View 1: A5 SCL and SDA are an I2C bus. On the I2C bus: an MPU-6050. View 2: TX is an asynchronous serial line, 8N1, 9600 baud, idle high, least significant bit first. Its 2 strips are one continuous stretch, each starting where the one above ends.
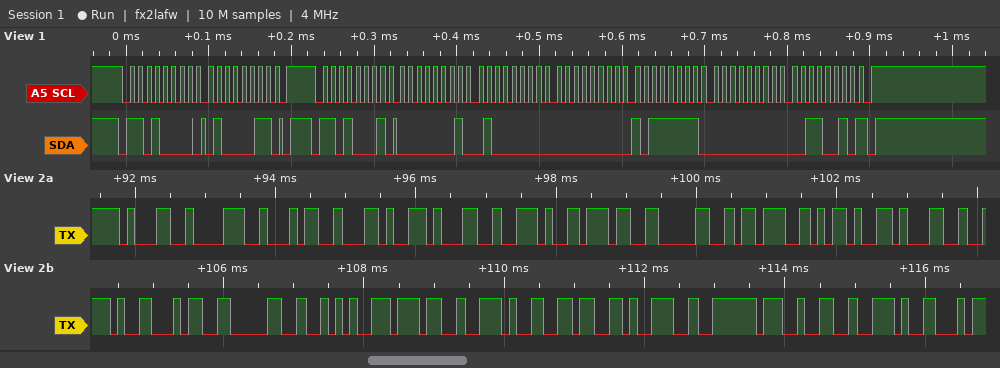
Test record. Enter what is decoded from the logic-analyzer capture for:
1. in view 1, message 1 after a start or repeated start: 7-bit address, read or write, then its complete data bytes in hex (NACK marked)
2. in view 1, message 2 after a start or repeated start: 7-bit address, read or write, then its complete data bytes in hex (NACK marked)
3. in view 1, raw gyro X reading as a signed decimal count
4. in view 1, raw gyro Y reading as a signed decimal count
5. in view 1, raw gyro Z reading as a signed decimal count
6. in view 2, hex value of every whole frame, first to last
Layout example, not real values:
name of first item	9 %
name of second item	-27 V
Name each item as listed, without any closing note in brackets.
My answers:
in view 1, message 1 after a start or repeated start: 7-bit address, read or write, then its complete data bytes in hex	0x68 write: 43
in view 1, message 2 after a start or repeated start: 7-bit address, read or write, then its complete data bytes in hex	0x68 read: 01 40 00 BF 00 32 NACK
in view 1, raw gyro X reading as a signed decimal count	320
in view 1, raw gyro Y reading as a signed decimal count	191
in view 1, raw gyro Z reading as a signed decimal count	50
in view 2, hex value of every whole frame, first to last	31 38 34 2C 31 2E 37 30 3B 2D 31 2E 34 30 2A 37 2E 36 39 7E 32 2E
